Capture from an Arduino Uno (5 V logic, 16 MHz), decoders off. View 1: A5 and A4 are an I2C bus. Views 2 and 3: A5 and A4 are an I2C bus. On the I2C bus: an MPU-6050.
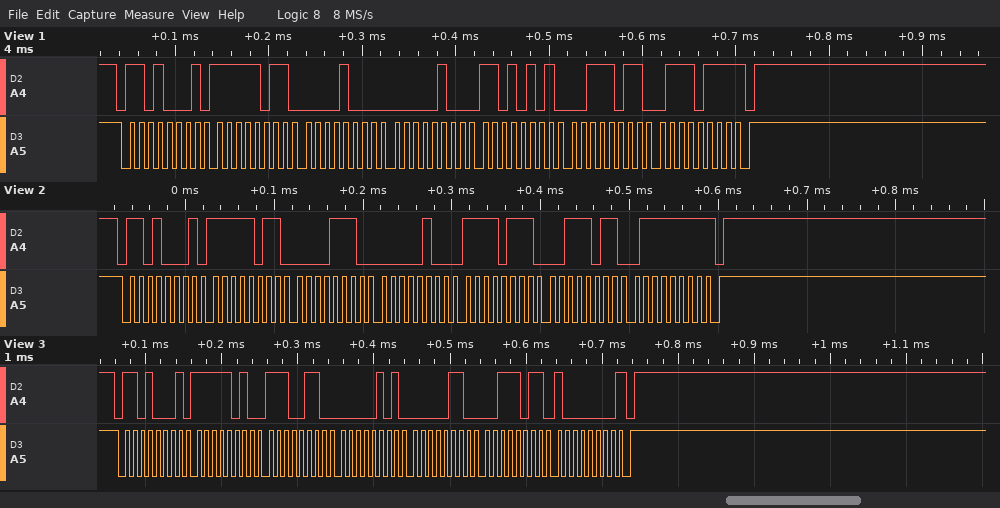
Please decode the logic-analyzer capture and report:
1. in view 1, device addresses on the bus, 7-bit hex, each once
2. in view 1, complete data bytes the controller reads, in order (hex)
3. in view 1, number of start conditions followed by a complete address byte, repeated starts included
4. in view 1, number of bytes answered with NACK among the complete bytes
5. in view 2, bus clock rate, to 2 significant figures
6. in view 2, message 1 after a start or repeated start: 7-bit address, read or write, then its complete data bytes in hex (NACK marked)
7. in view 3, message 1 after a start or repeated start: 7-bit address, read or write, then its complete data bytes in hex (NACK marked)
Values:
0x68
FB 08 04 D5 3B 77
1
1
100 kHz
0x68 read: FB 0E 04 F7 3B 7F NACK
0x68 read: FA E6 05 06 3B 80 NACK
